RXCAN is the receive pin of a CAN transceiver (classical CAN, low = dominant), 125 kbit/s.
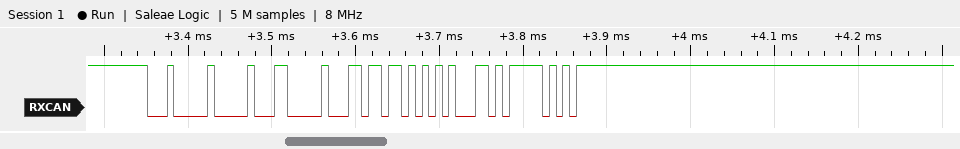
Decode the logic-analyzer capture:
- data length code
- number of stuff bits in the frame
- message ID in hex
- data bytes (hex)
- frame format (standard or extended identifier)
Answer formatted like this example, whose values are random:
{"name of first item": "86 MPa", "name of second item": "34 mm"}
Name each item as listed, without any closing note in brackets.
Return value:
{"data length code": "3", "number of stuff bits in the frame": "4", "message ID in hex": "0x100", "data bytes": "00 DB 55", "frame format": "standard"}
